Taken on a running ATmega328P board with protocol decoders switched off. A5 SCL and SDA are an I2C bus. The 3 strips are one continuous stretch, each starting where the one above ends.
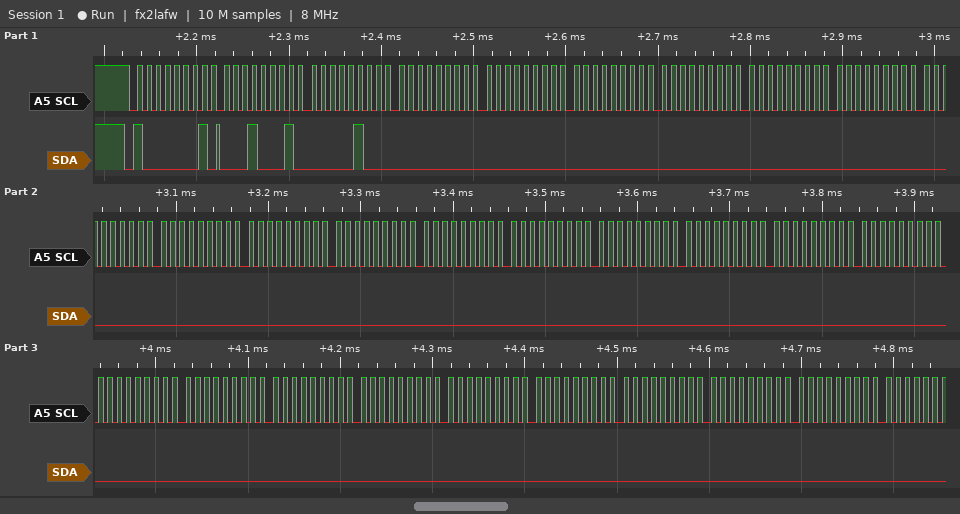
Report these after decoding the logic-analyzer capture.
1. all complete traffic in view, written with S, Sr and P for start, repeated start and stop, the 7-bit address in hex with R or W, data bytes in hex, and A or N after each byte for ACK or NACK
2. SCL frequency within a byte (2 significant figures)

S 40R A 11 A 04 A 00 A 00 A 00 A 00 A 00 A 00 A 00 A 00 A 00 A 00 A 00 A 00 A 00 A 00 A 00 A 00 A 00 A 00 A 00 A 00 A 00 A 00 A 00 A 00 A 00 A
100 kHz
